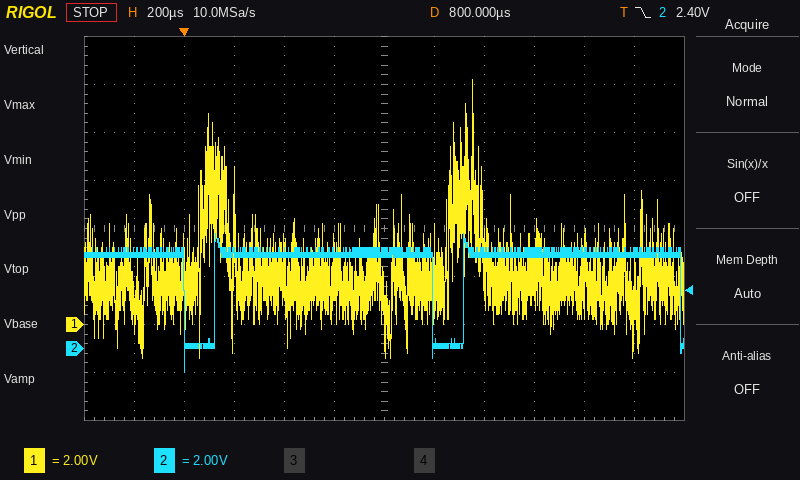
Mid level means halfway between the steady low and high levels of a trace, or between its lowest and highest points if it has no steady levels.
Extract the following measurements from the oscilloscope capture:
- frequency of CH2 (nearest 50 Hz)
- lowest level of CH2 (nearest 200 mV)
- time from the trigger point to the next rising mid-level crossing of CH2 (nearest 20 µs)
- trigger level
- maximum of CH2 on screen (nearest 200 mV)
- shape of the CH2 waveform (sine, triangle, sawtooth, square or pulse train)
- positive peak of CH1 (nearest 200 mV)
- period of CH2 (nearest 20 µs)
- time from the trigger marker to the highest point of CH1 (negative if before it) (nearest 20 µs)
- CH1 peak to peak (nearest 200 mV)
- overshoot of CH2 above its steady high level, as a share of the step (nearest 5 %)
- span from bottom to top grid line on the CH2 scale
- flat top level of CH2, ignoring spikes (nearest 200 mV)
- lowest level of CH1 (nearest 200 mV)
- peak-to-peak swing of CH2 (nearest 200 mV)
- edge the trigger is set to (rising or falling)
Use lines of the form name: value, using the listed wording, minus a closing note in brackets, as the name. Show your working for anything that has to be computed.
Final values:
frequency of CH2: 1 / 1.00 ms ≈ 1.00 kHz
lowest level of CH2: -1.0 V
time from the trigger point to the next rising mid-level crossing of CH2: 120 µs
trigger level: 2.40 V
maximum of CH2 on screen: 4.8 V
shape of the CH2 waveform: pulse train
positive peak of CH1: 10.2 V
period of CH2: 1.00 ms
time from the trigger marker to the highest point of CH1 (negative if before it): +1.16 ms
CH1 peak to peak: 10.2 V − (-1.4 V) = 11.6 V
overshoot of CH2 above its steady high level, as a share of the step: 20 %
span from bottom to top grid line on the CH2 scale: 16 V
flat top level of CH2, ignoring spikes: 4.0 V
lowest level of CH1: -1.4 V
peak-to-peak swing of CH2: 4.8 V − (-1.0 V) = 5.8 V
edge the trigger is set to: falling
